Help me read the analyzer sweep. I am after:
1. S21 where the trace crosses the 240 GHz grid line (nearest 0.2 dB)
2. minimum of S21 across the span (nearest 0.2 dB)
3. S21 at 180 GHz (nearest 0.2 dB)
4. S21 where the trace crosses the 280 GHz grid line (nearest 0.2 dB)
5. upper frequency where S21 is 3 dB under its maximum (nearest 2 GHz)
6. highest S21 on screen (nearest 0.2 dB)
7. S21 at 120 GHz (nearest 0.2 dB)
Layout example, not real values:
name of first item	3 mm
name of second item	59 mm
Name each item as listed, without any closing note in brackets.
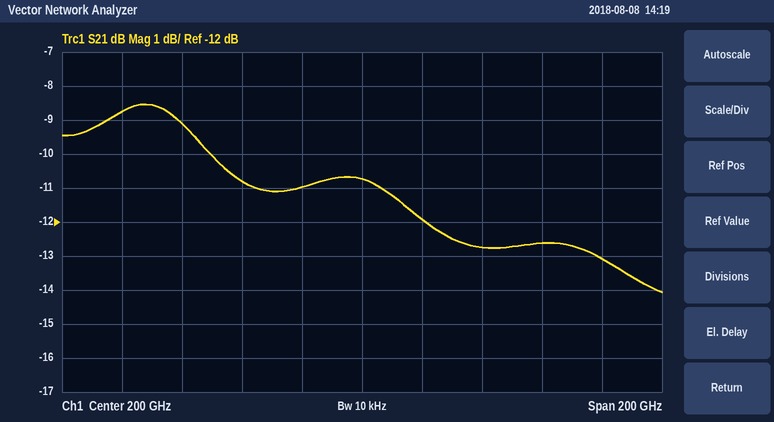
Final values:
S21 where the trace crosses the 240 GHz grid line	-12.8 dB
minimum of S21 across the span	-14.0 dB
S21 at 180 GHz	-11.0 dB
S21 where the trace crosses the 280 GHz grid line	-13.0 dB
upper frequency where S21 is 3 dB under its maximum	214 GHz
highest S21 on screen	-8.6 dB
S21 at 120 GHz	-8.8 dB
